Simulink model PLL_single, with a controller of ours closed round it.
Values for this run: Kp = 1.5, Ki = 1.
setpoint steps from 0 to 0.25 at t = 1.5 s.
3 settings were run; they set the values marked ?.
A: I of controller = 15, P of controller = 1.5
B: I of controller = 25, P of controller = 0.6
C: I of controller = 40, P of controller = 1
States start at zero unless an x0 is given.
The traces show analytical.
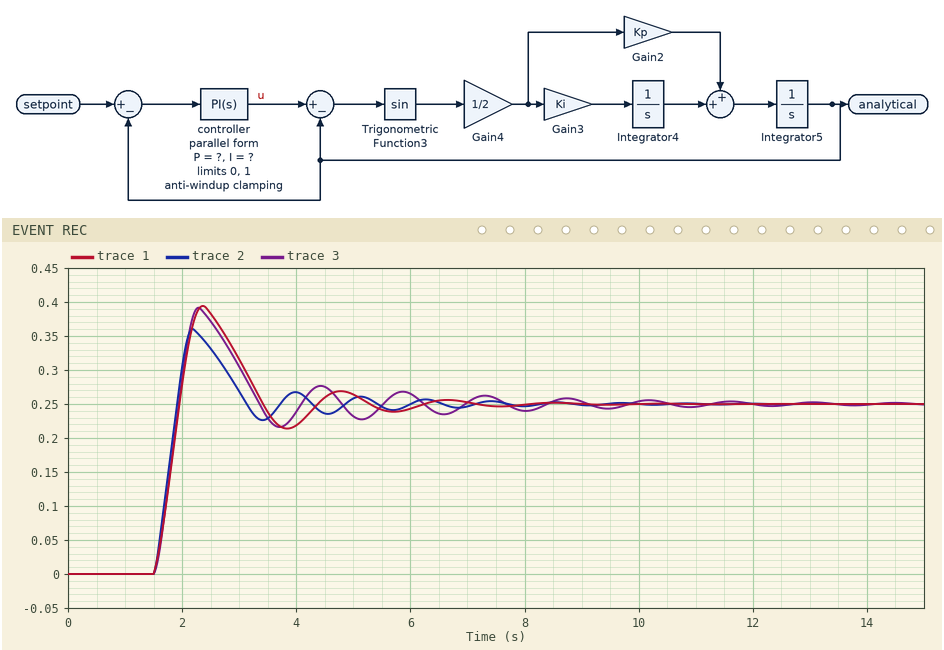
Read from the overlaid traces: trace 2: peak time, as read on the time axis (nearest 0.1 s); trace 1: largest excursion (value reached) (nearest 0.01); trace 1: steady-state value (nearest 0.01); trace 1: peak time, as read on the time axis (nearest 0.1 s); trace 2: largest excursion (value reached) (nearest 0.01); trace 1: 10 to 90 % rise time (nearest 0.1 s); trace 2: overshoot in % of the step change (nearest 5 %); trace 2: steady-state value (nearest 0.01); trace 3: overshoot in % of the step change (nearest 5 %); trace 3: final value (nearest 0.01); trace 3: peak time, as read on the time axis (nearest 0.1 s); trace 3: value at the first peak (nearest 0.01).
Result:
2.2 s
0.39
0.25
2.4 s
0.36
0.3 s
45 %
0.25
55 %
0.25
2.3 s
0.39
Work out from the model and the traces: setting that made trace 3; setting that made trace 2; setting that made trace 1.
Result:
B
C
A
